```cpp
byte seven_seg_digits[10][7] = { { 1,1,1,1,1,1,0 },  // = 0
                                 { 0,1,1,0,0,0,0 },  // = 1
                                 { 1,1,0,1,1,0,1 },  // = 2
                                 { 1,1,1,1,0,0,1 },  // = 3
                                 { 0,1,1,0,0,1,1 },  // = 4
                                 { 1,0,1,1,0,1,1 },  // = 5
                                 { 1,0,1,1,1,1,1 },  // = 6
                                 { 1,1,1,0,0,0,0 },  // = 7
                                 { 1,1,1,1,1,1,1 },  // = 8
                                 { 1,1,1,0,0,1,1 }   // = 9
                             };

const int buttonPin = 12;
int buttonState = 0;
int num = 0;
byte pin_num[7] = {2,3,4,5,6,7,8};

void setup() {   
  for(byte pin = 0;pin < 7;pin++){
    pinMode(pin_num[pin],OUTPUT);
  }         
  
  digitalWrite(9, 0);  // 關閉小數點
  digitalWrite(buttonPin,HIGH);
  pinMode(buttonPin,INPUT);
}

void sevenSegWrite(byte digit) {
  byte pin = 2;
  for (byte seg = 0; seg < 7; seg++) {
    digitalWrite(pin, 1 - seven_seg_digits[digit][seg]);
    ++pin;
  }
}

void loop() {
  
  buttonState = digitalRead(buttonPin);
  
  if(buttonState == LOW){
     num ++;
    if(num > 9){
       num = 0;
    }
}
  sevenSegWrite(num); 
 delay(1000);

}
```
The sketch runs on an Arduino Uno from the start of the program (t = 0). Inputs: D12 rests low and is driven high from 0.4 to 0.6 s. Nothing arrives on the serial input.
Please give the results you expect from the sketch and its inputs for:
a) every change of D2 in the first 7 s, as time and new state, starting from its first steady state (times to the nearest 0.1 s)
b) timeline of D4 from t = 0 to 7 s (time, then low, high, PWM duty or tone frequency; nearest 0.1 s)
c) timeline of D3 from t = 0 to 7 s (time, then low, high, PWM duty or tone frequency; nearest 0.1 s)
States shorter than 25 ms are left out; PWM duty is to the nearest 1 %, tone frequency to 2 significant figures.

0 s high; 1 s low; 3 s high; 4 s low
0 s low; 1 s high; 2 s low
0 s low; 4 s high; 6 s low
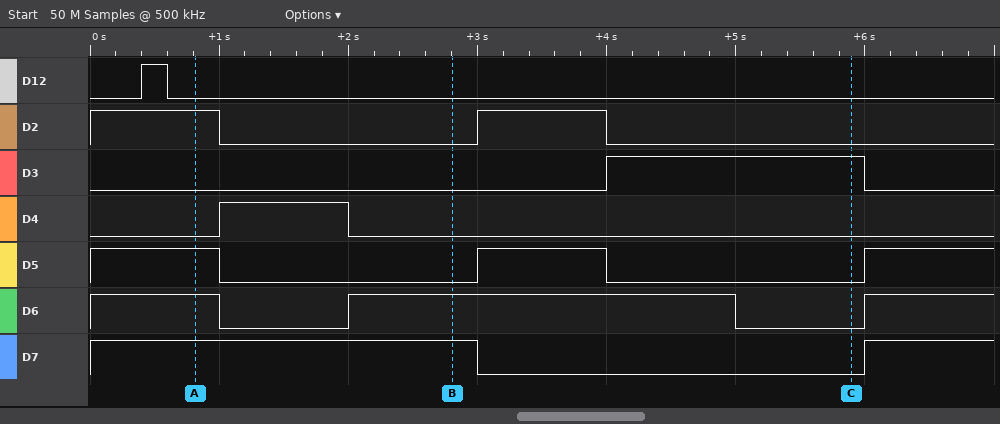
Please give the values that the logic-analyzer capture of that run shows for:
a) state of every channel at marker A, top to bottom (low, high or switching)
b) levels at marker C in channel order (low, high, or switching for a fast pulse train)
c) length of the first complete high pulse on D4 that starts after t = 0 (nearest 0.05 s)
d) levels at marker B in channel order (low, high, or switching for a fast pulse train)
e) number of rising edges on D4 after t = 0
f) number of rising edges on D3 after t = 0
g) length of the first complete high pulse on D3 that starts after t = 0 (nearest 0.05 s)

D12 low, D2 high, D3 low, D4 low, D5 high, D6 high, D7 high
D12 low, D2 low, D3 high, D4 low, D5 low, D6 low, D7 low
1.00 s
D12 low, D2 low, D3 low, D4 low, D5 low, D6 high, D7 high
1
1
2.00 s
